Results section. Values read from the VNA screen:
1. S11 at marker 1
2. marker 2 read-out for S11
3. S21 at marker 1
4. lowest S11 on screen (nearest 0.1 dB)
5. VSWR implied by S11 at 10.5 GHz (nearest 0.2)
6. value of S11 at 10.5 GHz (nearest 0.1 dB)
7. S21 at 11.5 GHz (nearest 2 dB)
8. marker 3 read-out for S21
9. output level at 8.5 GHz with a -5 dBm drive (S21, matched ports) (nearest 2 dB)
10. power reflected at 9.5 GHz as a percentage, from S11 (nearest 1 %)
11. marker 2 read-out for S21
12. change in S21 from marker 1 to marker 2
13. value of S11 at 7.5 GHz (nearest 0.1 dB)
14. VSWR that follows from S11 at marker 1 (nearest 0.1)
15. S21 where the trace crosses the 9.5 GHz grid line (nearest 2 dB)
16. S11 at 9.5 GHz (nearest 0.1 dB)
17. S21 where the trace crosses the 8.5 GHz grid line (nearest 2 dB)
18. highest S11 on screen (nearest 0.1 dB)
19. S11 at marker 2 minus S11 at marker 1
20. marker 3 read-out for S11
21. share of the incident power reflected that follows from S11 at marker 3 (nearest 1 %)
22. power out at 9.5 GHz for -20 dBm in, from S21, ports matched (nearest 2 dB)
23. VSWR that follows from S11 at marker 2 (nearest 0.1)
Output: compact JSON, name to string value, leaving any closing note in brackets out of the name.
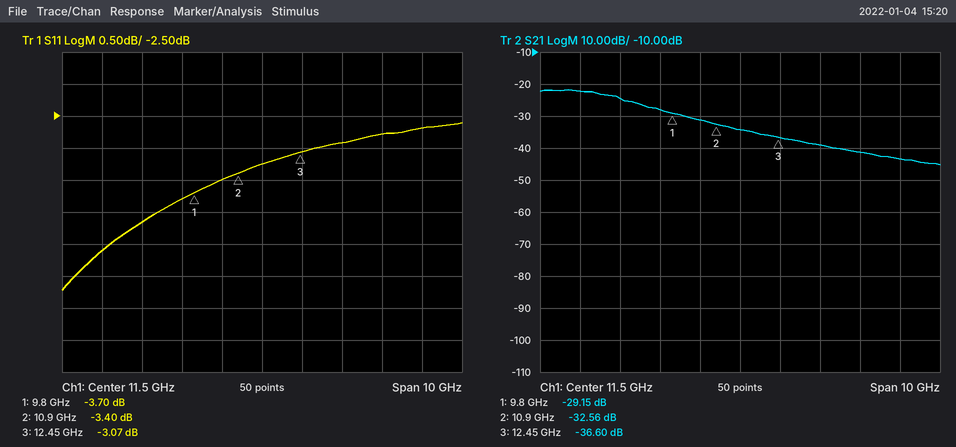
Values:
{"S11 at marker 1": "-3.70 dB", "marker 2 read-out for S11": "-3.40 dB", "S21 at marker 1": "-29.15 dB", "lowest S11 on screen": "-5.2 dB", "VSWR implied by S11 at 10.5 GHz": "5.0", "value of S11 at 10.5 GHz": "-3.5 dB", "S21 at 11.5 GHz": "-34 dB", "marker 3 read-out for S21": "-36.60 dB", "output level at 8.5 GHz with a -5 dBm drive (S21, matched ports)": "-30 dBm", "power reflected at 9.5 GHz as a percentage, from S11": "42 %", "marker 2 read-out for S21": "-32.56 dB", "change in S21 from marker 1 to marker 2": "-3.41 dB", "value of S11 at 7.5 GHz": "-4.6 dB", "VSWR that follows from S11 at marker 1": "4.8", "S21 where the trace crosses the 9.5 GHz grid line": "-28 dB", "S11 at 9.5 GHz": "-3.8 dB", "S21 where the trace crosses the 8.5 GHz grid line": "-24 dB", "highest S11 on screen": "-2.6 dB", "S11 at marker 2 minus S11 at marker 1": "0.30 dB", "marker 3 read-out for S11": "-3.07 dB", "share of the incident power reflected that follows from S11 at marker 3": "49 %", "power out at 9.5 GHz for -20 dBm in, from S21, ports matched": "-48 dBm", "VSWR that follows from S11 at marker 2": "5.2"}
